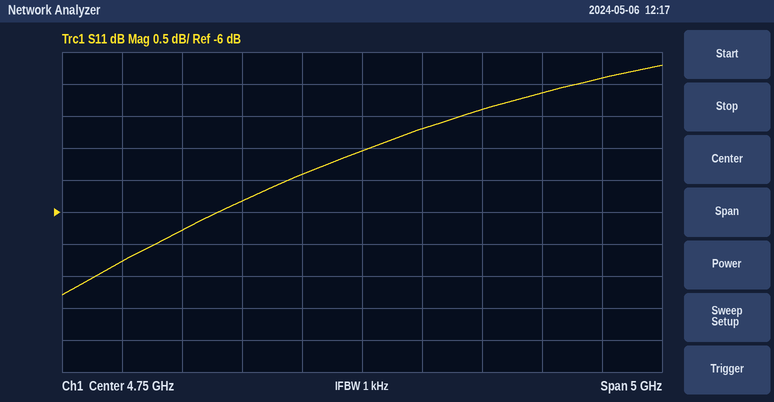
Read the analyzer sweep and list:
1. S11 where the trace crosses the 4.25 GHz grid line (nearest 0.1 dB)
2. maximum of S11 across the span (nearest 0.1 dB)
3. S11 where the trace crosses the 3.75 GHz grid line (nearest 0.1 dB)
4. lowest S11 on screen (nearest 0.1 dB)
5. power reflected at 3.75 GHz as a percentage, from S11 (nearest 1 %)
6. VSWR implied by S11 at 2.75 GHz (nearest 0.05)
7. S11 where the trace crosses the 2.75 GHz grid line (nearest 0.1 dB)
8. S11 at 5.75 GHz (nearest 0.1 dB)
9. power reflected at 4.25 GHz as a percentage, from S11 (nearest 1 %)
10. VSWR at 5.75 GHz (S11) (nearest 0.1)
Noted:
-5.4 dB
-3.7 dB
-5.8 dB
-7.3 dB
26 %
2.70
-6.8 dB
-4.4 dB
29 %
4.0
